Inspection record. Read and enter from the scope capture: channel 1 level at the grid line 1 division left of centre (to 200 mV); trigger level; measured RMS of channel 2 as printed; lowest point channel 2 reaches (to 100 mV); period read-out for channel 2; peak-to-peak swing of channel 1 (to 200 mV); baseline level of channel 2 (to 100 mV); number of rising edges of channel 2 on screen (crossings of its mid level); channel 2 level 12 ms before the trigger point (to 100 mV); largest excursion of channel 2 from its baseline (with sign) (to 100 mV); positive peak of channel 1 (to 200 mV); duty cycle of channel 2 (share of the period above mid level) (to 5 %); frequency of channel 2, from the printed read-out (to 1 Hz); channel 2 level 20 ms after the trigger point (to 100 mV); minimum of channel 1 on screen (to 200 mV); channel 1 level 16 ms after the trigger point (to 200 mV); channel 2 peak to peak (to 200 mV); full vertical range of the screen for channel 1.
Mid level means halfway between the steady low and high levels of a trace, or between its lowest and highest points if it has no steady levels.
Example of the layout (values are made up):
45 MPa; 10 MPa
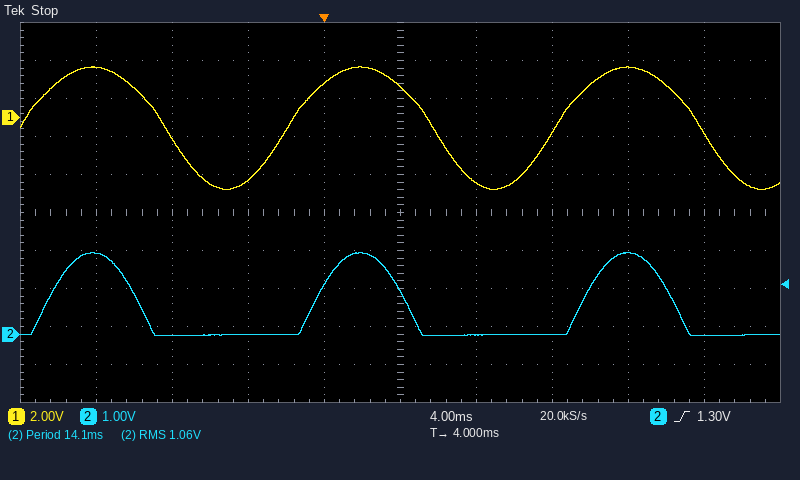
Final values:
1.8 V; 1.30 V; 1.06 V; 0.0 V; 14.1 ms; 6.4 V; 0.0 V; 3; 2.1 V; +2.2 V; 2.6 V; 30 %; 71 Hz; 0.0 V; -3.8 V; 2.6 V; 2.2 V; 20 V
